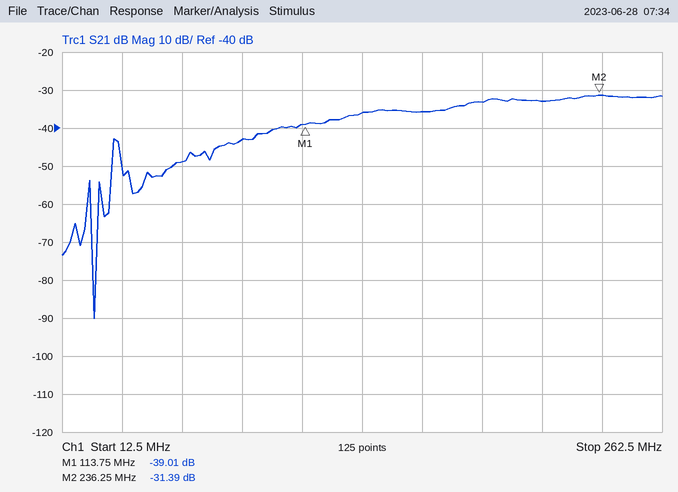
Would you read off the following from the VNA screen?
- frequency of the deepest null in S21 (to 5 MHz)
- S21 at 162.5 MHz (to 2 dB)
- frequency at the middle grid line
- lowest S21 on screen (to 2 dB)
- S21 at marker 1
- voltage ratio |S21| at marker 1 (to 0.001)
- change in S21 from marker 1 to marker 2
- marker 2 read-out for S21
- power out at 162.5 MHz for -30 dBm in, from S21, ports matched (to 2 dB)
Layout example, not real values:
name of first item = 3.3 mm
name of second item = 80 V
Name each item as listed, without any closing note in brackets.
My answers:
frequency of the deepest null in S21 = 25 MHz
S21 at 162.5 MHz = -36 dB
frequency at the middle grid line = 137.5 MHz
lowest S21 on screen = -90 dB
S21 at marker 1 = -39.01 dB
voltage ratio |S21| at marker 1 = 0.011
change in S21 from marker 1 to marker 2 = 7.62 dB
marker 2 read-out for S21 = -31.39 dB
power out at 162.5 MHz for -30 dBm in, from S21, ports matched = -66 dBm
